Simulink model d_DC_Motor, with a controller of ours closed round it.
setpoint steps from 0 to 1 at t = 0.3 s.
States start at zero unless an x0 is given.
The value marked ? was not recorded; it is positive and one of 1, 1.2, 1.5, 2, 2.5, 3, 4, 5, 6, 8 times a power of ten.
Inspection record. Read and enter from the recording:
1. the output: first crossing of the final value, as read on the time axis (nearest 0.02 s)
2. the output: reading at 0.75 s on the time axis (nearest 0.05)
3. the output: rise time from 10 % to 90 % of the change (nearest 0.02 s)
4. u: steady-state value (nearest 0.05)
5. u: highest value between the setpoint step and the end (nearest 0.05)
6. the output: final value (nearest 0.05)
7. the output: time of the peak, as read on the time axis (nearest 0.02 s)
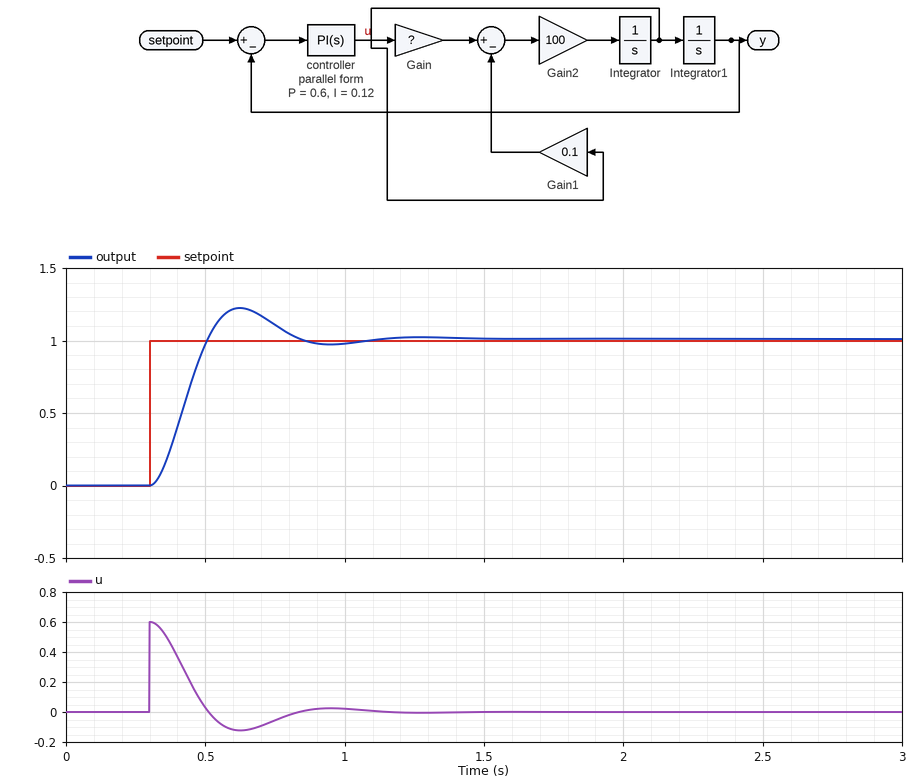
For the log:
0.50 s
1.10
0.14 s
0.00
0.60
1.00
0.62 s
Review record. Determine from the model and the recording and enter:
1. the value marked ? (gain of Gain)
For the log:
2
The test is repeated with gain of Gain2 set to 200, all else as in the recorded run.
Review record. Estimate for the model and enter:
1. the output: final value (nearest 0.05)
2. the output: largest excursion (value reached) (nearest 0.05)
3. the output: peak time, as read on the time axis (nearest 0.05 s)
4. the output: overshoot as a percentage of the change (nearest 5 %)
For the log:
1.00
1.10
0.55 s
10 %
